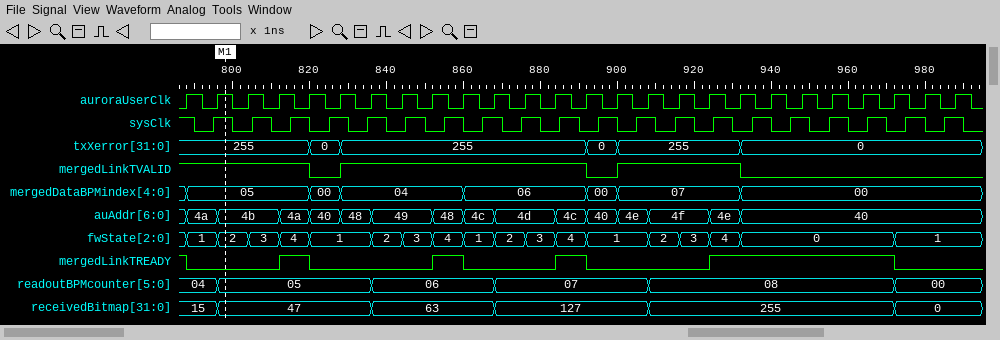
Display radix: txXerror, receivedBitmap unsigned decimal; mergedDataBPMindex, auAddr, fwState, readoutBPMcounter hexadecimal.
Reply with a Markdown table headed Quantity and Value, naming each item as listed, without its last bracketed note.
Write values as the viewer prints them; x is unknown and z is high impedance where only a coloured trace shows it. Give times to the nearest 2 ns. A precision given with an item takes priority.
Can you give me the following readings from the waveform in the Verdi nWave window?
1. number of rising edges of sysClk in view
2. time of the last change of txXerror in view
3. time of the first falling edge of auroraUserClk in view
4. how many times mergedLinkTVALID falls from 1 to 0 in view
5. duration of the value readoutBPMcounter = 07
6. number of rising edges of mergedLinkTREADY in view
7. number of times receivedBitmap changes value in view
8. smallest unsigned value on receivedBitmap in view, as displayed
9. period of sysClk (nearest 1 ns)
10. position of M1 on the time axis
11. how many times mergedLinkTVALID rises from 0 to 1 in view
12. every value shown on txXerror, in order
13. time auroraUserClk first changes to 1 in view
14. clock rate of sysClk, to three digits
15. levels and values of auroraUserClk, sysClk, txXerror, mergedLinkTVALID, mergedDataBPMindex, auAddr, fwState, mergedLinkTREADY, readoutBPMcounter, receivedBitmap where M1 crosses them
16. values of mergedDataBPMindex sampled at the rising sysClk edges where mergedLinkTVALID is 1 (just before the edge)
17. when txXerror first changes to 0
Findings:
| Quantity | Value |
|---|---|
| number of rising edges of sysClk in view | 20 |
| time of the last change of txXerror in view | 932 ns |
| time of the first falling edge of auroraUserClk in view | 792 ns |
| how many times mergedLinkTVALID falls from 1 to 0 in view | 3 |
| duration of the value readoutBPMcounter = 07 | 40 ns |
| number of rising edges of mergedLinkTREADY in view | 4 |
| number of times receivedBitmap changes value in view | 5 |
| smallest unsigned value on receivedBitmap in view, as displayed | 0 |
| period of sysClk | 10 ns |
| position of M1 on the time axis | 798 ns |
| how many times mergedLinkTVALID rises from 0 to 1 in view | 2 |
| every value shown on txXerror, in order | 255, 0, 255, 0, 255, 0 |
| time auroraUserClk first changes to 1 in view | 788 ns |
| clock rate of sysClk, to three digits | 100 MHz |
| levels and values of auroraUserClk, sysClk, txXerror, mergedLinkTVALID, mergedDataBPMindex, auAddr, fwState, mergedLinkTREADY, readoutBPMcounter, receivedBitmap where M1 crosses them | auroraUserClk=1, sysClk=1, txXerror=255, mergedLinkTVALID=1, mergedDataBPMindex=05, auAddr=4b, fwState=2, mergedLinkTREADY=0, readoutBPMcounter=05, receivedBitmap=47 |
| values of mergedDataBPMindex sampled at the rising sysClk edges where mergedLinkTVALID is 1 | 05, 05, 05, 04, 04, 04, 06, 06, 06, 07, 07, 07 |
| when txXerror first changes to 0 | 820 ns |
